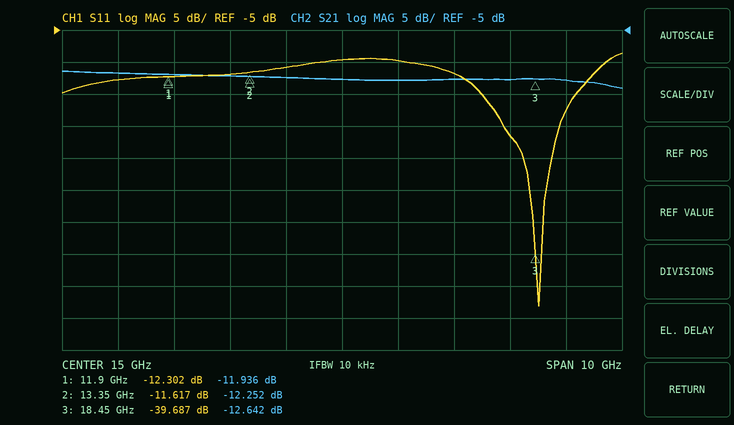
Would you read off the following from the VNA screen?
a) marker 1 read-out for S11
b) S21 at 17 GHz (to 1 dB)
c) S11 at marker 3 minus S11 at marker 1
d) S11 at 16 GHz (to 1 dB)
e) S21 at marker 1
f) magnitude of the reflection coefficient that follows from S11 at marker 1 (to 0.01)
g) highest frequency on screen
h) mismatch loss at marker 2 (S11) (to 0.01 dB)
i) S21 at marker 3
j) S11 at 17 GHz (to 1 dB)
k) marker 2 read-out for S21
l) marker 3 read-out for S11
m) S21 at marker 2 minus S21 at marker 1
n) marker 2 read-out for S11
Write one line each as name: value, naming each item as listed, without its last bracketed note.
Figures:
marker 1 read-out for S11: -12.302 dB
S21 at 17 GHz: -13 dB
S11 at marker 3 minus S11 at marker 1: -27.385 dB
S11 at 16 GHz: -10 dB
S21 at marker 1: -11.936 dB
magnitude of the reflection coefficient that follows from S11 at marker 1: 0.24
highest frequency on screen: 20 GHz
mismatch loss at marker 2 (S11): 0.31 dB
S21 at marker 3: -12.642 dB
S11 at 17 GHz: -12 dB
marker 2 read-out for S21: -12.252 dB
marker 3 read-out for S11: -39.687 dB
S21 at marker 2 minus S21 at marker 1: -0.316 dB
marker 2 read-out for S11: -11.617 dB
